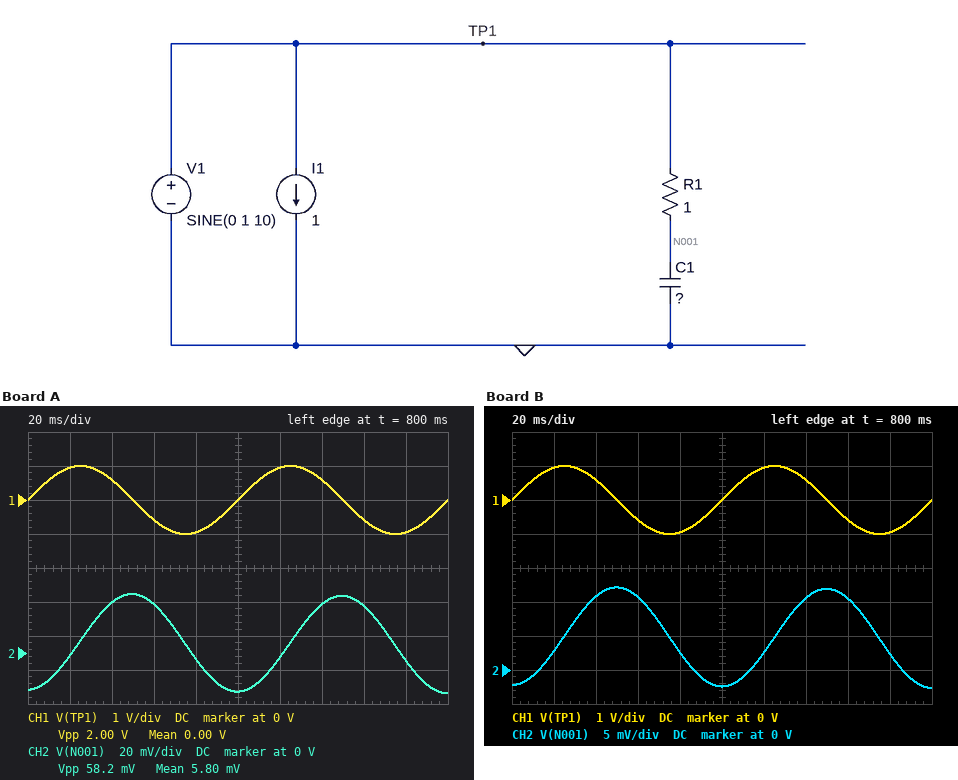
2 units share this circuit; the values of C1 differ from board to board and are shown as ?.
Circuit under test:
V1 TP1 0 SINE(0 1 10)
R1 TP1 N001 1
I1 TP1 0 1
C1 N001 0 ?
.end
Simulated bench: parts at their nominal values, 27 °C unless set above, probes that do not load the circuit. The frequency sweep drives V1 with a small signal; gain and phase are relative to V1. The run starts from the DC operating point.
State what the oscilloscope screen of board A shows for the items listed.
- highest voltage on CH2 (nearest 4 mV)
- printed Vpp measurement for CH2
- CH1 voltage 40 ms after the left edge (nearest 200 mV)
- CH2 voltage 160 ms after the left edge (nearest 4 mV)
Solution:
36 mV
58.2 mV
600 mV
28 mV
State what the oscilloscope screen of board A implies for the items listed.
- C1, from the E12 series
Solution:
560 mF
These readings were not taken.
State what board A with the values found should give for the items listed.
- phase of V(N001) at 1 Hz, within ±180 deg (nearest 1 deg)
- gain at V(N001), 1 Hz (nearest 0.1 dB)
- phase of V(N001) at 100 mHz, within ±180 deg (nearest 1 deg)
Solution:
-74 deg
-11.3 dB
-19 deg
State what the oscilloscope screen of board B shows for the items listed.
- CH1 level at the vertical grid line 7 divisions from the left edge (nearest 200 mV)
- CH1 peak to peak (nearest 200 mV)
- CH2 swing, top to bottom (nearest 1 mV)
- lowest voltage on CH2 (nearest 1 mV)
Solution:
600 mV
2.0 V
15 mV
-3 mV
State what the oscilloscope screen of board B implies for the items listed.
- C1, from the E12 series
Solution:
2.2 F
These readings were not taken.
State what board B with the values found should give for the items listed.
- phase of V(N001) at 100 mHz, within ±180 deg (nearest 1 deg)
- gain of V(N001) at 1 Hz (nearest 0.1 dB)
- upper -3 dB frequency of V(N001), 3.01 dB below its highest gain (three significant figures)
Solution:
-54 deg
-22.8 dB
72.3 mHz
